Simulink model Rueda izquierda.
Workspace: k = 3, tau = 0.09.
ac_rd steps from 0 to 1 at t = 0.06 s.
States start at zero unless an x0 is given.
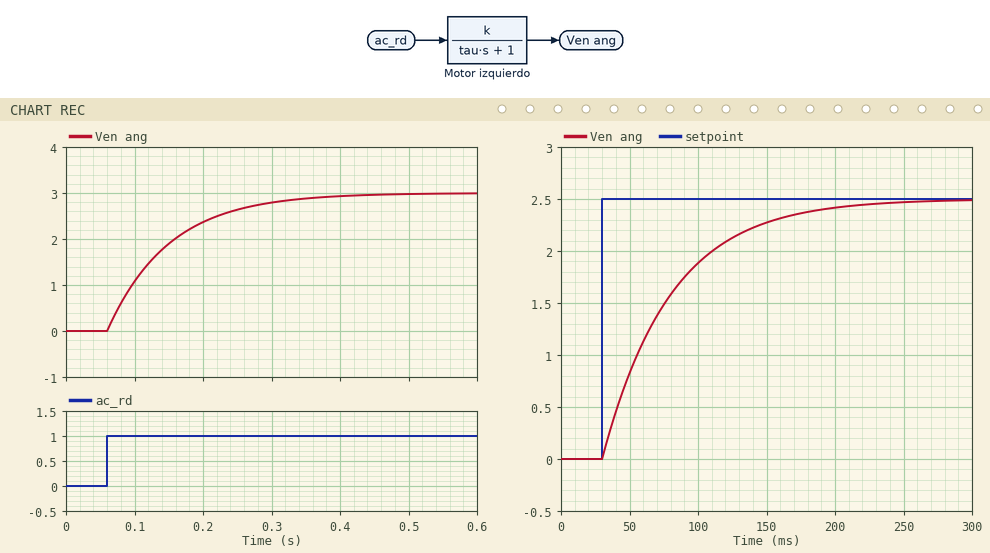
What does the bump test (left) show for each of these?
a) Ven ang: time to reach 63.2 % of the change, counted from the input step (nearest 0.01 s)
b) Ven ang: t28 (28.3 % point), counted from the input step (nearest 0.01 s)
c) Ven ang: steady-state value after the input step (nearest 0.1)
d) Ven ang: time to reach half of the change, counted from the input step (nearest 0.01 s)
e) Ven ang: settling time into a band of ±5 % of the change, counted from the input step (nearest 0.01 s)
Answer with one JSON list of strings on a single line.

["0.09 s", "0.03 s", "3.0", "0.06 s", "0.27 s"]
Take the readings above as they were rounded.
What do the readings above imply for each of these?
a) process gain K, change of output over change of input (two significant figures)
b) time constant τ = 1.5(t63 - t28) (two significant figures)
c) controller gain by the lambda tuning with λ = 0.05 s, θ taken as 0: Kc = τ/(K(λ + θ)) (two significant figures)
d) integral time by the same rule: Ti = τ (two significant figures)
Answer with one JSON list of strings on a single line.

["3.0", "0.090 s", "0.60", "0.090 s"]
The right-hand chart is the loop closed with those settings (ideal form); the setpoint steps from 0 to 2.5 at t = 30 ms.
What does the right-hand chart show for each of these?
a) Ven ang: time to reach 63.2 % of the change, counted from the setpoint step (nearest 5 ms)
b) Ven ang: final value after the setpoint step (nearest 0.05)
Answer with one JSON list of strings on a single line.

["50 ms", "2.50"]
